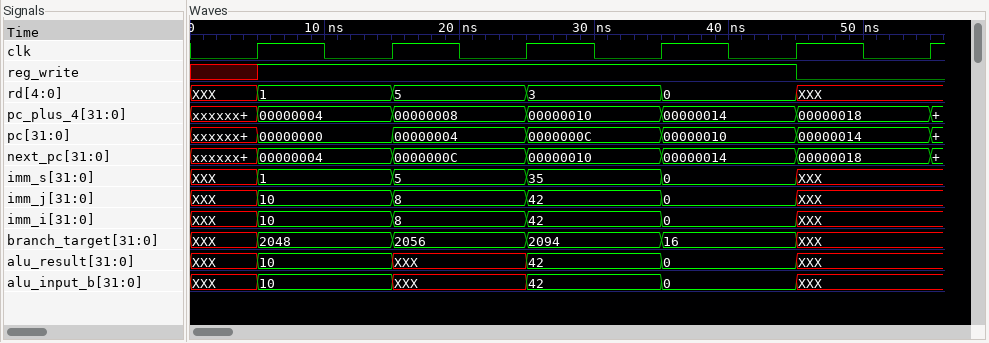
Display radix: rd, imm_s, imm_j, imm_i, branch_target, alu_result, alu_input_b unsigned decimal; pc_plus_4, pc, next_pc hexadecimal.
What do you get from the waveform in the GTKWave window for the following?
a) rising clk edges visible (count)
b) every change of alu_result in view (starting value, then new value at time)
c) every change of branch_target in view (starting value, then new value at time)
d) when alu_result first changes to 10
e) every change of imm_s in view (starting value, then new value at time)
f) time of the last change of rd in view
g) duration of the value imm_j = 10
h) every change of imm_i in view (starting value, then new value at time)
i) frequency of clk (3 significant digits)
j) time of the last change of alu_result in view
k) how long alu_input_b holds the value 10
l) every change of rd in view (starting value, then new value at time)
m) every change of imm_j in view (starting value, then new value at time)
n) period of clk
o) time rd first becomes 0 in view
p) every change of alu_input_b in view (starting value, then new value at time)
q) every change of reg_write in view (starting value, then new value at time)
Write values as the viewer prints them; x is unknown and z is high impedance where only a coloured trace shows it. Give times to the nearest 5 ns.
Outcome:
6
XXX, 10 at 5 ns, XXX at 15 ns, 42 at 25 ns, 0 at 35 ns, XXX at 45 ns
XXX, 2048 at 5 ns, 2056 at 15 ns, 2094 at 25 ns, 16 at 35 ns, XXX at 45 ns
5 ns
XXX, 1 at 5 ns, 5 at 15 ns, 35 at 25 ns, 0 at 35 ns, XXX at 45 ns
45 ns
10 ns
XXX, 10 at 5 ns, 8 at 15 ns, 42 at 25 ns, 0 at 35 ns, XXX at 45 ns
100 MHz
45 ns
10 ns
XXX, 1 at 5 ns, 5 at 15 ns, 3 at 25 ns, 0 at 35 ns, XXX at 45 ns
XXX, 10 at 5 ns, 8 at 15 ns, 42 at 25 ns, 0 at 35 ns, XXX at 45 ns
10 ns
35 ns
XXX, 10 at 5 ns, XXX at 15 ns, 42 at 25 ns, 0 at 35 ns, XXX at 45 ns
x, 1 at 5 ns, 0 at 45 ns
